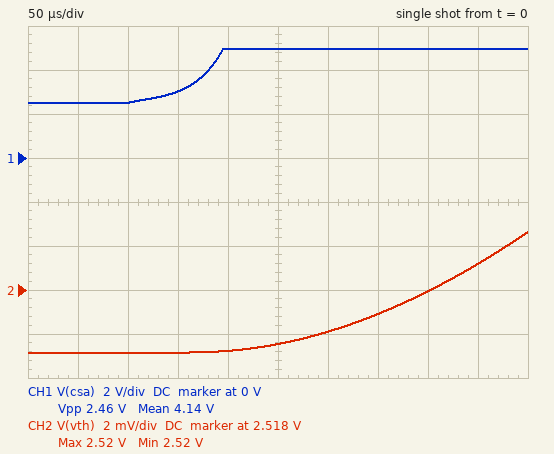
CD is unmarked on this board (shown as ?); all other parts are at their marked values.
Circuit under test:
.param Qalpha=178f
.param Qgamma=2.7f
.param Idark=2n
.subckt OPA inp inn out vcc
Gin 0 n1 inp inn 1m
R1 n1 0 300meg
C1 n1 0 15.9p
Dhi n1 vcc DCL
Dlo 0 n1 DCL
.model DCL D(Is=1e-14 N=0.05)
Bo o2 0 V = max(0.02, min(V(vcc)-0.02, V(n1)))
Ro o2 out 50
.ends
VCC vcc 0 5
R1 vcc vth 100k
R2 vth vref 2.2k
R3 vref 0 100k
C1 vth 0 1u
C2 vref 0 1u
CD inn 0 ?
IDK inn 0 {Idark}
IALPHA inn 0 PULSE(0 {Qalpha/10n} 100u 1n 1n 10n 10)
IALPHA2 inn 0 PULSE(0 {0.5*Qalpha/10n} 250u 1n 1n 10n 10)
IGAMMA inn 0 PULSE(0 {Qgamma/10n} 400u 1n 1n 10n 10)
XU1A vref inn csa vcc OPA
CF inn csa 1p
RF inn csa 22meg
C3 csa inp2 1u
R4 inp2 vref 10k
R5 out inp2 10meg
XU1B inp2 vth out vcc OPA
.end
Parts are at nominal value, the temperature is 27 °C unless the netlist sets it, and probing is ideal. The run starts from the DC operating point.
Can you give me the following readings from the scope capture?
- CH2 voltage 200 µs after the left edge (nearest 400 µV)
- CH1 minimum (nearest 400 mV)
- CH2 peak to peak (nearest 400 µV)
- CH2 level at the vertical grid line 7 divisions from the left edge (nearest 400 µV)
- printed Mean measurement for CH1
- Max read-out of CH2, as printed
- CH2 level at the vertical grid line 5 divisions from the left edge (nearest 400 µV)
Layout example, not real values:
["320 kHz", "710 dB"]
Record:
["2.5152 V", "2.4 V", "5.6 mV", "2.5168 V", "4.14 V", "2.52 V", "2.5156 V"]
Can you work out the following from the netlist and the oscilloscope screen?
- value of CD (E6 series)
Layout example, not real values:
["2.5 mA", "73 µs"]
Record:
["1 nF"]
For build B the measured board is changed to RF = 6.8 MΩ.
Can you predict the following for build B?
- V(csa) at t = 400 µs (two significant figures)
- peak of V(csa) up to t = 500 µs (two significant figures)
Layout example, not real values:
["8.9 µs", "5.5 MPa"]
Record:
["2.5 V", "2.6 V"]
